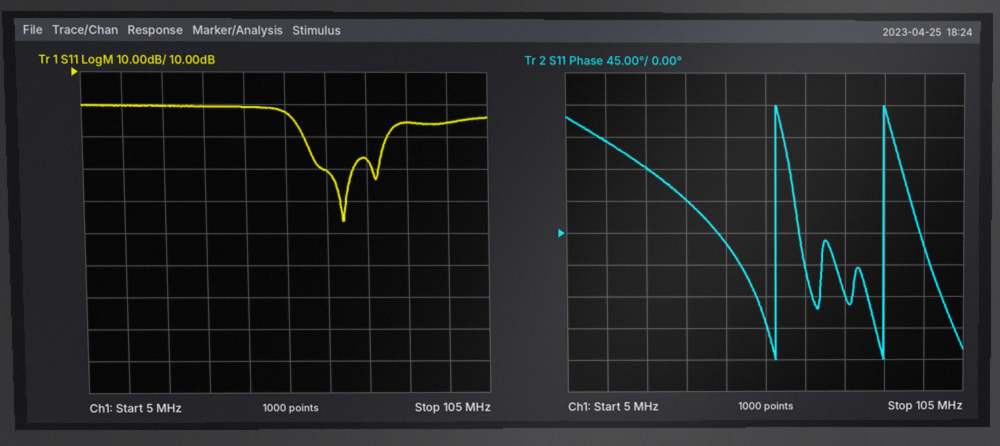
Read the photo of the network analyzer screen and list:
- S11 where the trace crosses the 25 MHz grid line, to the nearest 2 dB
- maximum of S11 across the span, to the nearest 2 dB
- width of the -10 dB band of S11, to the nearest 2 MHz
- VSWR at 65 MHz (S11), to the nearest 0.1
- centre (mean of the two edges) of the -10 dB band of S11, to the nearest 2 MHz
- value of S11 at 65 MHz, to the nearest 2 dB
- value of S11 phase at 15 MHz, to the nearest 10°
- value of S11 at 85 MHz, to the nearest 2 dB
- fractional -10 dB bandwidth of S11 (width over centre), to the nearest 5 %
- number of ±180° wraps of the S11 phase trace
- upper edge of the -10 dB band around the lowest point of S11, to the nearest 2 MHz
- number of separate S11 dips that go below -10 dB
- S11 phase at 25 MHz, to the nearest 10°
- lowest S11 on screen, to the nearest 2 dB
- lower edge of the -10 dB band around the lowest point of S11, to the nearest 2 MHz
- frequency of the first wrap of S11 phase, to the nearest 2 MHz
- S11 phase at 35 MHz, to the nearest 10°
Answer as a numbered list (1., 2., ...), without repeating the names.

1. 0 dB
2. 0 dB
3. 20 MHz
4. 1.2
5. 70 MHz
6. -20 dB
7. 130°
8. -6 dB
9. 30 %
10. 2
11. 80 MHz
12. 2
13. 90°
14. -36 dB
15. 60 MHz
16. 58 MHz
17. 50°
